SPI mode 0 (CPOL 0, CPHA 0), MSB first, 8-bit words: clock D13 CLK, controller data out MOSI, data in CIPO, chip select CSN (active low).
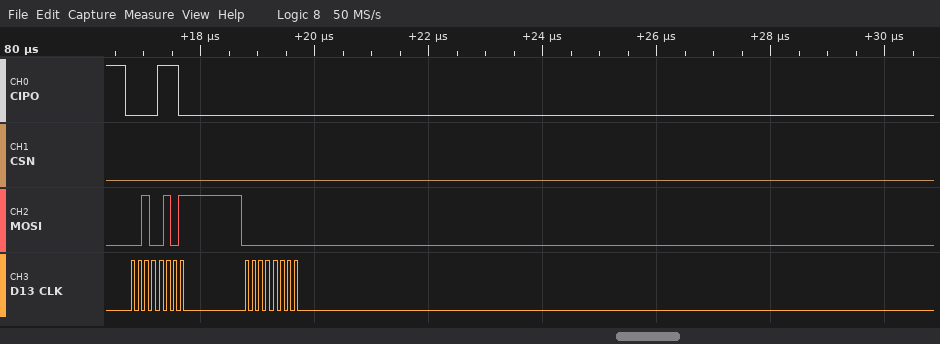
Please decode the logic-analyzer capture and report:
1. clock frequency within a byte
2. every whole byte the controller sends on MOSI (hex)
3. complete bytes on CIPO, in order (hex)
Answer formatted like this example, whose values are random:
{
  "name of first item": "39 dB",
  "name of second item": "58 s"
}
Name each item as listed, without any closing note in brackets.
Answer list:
{
  "clock frequency within a byte": "8 MHz",
  "every whole byte the controller sends on MOSI": "0x25 0x00",
  "complete bytes on CIPO, in order": "0x0E 0x00"
}
